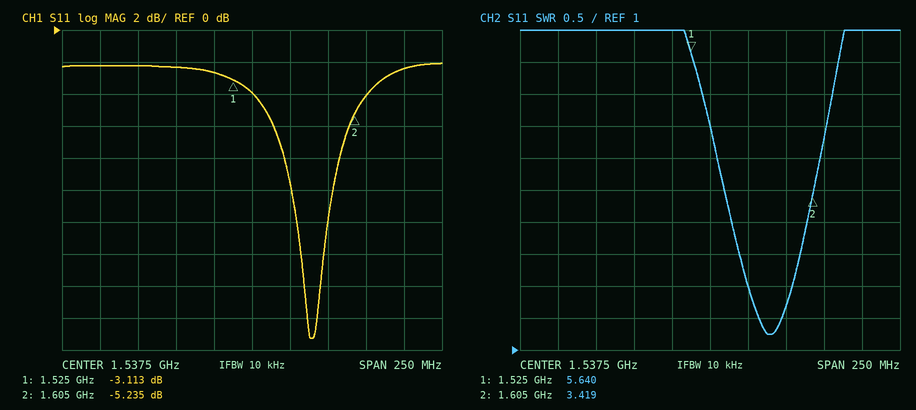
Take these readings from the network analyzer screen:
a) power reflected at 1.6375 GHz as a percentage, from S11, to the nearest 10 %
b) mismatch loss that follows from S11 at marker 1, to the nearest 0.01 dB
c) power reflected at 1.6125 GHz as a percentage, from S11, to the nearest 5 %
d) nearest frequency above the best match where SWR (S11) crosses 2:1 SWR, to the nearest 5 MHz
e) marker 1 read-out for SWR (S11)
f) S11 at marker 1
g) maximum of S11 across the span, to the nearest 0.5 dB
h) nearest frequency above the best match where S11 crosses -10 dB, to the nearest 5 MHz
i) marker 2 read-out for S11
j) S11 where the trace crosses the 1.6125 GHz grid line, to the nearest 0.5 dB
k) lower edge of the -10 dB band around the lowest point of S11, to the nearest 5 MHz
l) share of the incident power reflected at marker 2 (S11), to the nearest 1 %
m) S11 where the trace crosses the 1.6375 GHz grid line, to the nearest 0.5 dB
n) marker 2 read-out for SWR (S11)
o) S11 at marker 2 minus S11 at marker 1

60 %
2.91 dB
40 %
1.590 GHz
5.640
-3.113 dB
-2.0 dB
1.590 GHz
-5.235 dB
-4.0 dB
1.565 GHz
30 %
-2.5 dB
3.419
-2.122 dB
